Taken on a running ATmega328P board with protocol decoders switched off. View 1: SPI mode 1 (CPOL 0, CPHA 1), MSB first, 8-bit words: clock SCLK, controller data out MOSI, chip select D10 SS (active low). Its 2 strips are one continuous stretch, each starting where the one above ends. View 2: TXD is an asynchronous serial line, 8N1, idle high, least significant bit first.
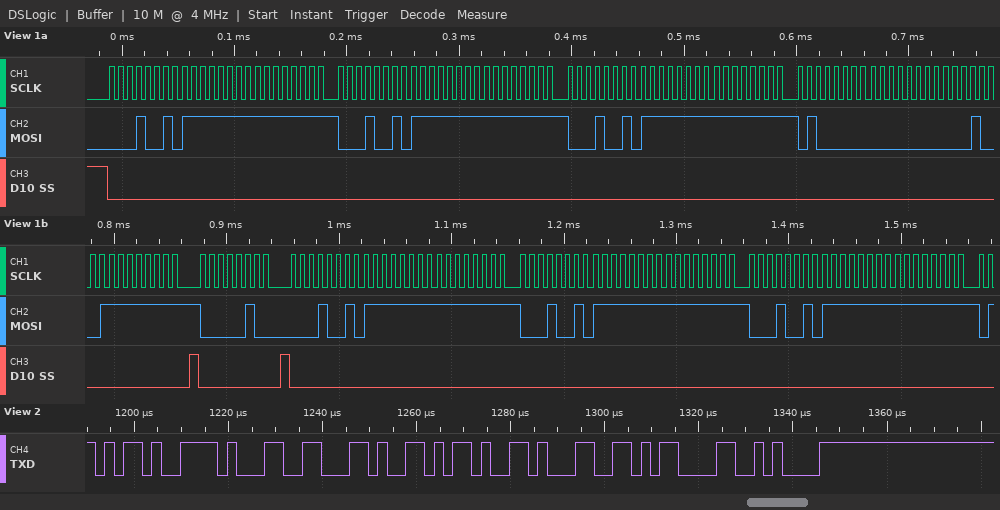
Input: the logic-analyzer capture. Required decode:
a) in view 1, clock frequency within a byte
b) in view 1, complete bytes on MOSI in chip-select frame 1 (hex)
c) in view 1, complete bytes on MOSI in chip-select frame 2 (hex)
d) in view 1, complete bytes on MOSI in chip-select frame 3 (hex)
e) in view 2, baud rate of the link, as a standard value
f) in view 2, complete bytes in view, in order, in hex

125 kHz
12 FF FF 12 FF FF 12 FF FF 40 00 11 FF
04
12 FF FF 12 FF FF 12 FF FF
500000 baud
2D 31 2C 2D 31 0D 0A
